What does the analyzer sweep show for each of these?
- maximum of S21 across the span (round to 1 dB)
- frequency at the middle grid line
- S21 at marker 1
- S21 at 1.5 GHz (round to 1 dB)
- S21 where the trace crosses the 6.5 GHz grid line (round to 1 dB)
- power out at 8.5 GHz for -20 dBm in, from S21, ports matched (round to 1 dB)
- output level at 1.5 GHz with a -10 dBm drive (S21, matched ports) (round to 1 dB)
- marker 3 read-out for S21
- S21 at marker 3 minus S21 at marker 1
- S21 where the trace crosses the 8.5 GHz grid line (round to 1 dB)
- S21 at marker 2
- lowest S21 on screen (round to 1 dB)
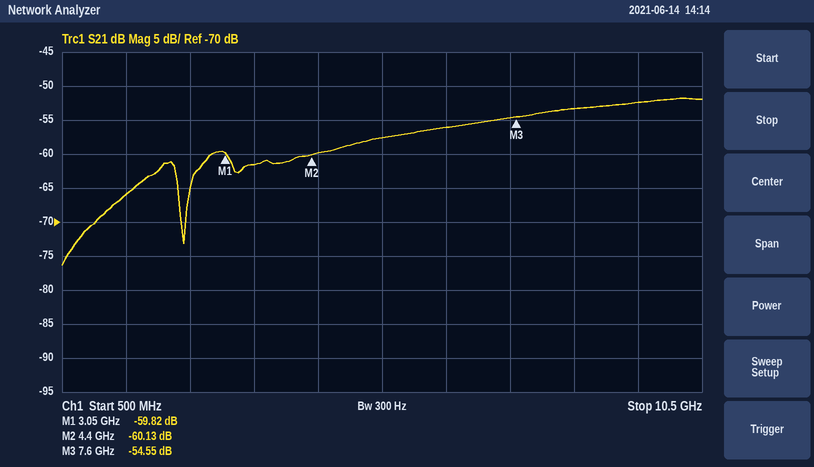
-52 dB
5.5 GHz
-59.82 dB
-66 dB
-56 dB
-73 dBm
-76 dBm
-54.55 dB
5.27 dB
-53 dB
-60.13 dB
-76 dB
